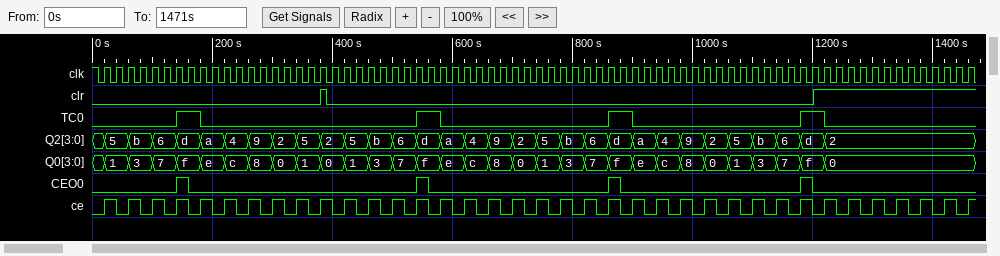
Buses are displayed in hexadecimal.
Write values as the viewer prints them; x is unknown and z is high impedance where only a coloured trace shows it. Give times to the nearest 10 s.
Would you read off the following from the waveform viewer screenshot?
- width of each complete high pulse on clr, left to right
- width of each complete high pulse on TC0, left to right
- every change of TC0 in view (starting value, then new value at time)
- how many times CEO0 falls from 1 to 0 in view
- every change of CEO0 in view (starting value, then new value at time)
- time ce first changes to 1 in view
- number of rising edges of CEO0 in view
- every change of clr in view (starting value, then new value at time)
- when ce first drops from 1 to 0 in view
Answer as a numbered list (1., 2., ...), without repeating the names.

1. 10 s
2. 40 s, 40 s, 40 s, 40 s
3. 0, 1 at 140 s, 0 at 180 s, 1 at 540 s, 0 at 580 s, 1 at 860 s, 0 at 900 s, 1 at 1180 s, 0 at 1220 s
4. 4
5. 0, 1 at 140 s, 0 at 160 s, 1 at 540 s, 0 at 560 s, 1 at 860 s, 0 at 880 s, 1 at 1180 s, 0 at 1200 s
6. 20 s
7. 4
8. 0, 1 at 380 s, 0 at 390 s, 1 at 1200 s
9. 40 s
